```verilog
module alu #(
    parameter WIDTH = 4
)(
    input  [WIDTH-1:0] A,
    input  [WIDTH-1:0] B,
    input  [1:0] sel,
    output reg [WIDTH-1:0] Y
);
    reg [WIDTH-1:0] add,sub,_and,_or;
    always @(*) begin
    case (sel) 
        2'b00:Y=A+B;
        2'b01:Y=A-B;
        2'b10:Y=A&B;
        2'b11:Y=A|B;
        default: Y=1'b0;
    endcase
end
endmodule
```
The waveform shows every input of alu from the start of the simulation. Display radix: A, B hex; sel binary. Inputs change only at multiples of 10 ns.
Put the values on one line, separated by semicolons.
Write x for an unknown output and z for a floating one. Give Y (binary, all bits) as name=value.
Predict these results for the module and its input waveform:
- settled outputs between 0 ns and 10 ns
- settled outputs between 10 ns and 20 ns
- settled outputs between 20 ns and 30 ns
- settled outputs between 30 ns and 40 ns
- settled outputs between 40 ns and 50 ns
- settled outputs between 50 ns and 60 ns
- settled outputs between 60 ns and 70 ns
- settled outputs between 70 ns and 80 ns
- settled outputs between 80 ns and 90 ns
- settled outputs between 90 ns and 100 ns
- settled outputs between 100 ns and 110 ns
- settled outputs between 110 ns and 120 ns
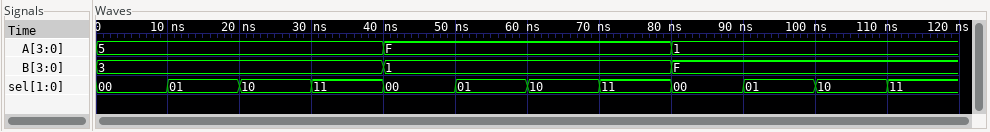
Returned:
Y=1000; Y=0010; Y=0001; Y=0111; Y=0000; Y=1110; Y=0001; Y=1111; Y=0000; Y=0010; Y=0001; Y=1111
